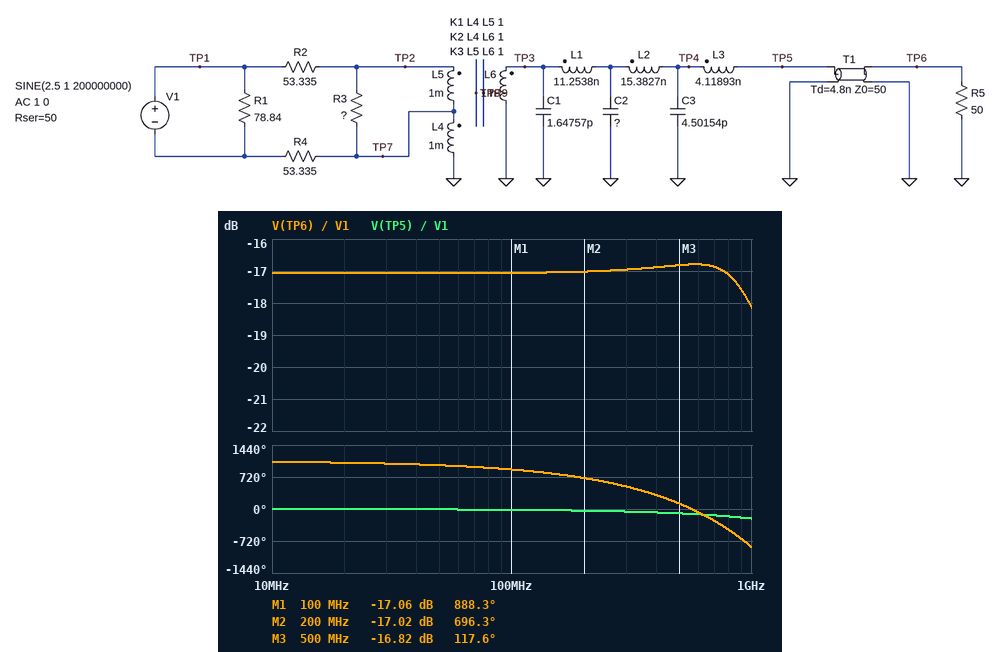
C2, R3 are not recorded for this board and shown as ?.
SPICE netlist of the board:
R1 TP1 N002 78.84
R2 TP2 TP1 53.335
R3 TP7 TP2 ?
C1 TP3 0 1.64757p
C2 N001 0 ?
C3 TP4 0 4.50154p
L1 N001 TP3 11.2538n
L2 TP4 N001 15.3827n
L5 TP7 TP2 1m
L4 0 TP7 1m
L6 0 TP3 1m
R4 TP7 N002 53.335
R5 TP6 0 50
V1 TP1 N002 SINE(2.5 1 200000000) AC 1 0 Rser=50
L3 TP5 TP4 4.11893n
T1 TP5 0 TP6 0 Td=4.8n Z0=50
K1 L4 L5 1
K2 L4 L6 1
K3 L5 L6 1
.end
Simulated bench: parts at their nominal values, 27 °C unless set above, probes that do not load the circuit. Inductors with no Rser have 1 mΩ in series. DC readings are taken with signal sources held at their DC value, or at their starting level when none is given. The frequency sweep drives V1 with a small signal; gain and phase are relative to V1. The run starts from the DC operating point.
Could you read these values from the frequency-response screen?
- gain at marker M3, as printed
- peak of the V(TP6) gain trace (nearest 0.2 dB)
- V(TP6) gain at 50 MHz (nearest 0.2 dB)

-16.82 dB
-16.8 dB
-17.0 dB
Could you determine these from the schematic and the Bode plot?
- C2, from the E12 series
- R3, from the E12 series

3.3 pF
220 Ω
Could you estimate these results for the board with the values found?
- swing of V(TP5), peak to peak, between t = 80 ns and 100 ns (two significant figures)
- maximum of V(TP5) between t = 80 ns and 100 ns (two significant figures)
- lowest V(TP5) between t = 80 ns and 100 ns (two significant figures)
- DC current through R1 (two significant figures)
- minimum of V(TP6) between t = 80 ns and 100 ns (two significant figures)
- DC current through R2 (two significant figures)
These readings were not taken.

280 mV
140 mV
-140 mV
15 mA
-140 mV
11 mA
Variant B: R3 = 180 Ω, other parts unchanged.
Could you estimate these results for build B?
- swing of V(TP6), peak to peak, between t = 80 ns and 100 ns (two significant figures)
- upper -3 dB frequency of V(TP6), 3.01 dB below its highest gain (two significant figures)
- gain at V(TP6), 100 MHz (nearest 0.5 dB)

270 mV
1.3 GHz
-17.5 dB
